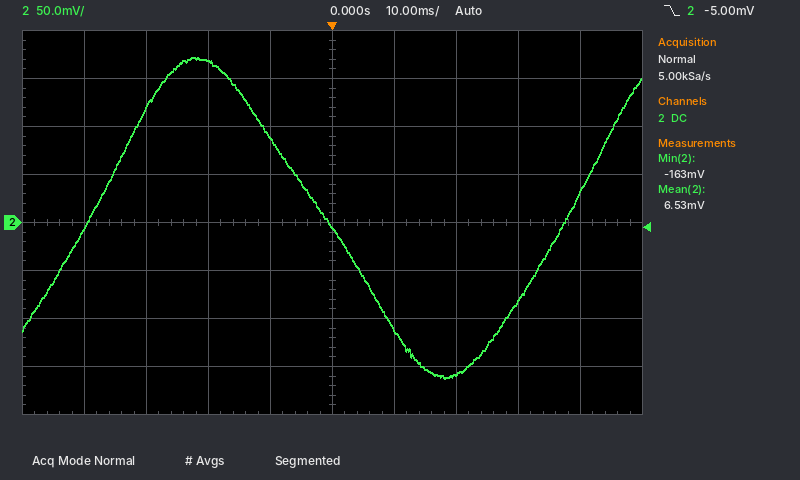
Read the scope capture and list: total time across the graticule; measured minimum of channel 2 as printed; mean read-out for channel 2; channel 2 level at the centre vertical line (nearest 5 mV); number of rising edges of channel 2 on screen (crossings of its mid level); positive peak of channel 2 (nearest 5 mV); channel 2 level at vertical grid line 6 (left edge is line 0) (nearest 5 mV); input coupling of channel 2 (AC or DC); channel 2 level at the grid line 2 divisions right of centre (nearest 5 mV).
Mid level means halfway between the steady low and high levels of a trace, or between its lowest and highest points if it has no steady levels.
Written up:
100 ms
-163 mV
6.53 mV
-5 mV
2
170 mV
-110 mV
DC
-160 mV
